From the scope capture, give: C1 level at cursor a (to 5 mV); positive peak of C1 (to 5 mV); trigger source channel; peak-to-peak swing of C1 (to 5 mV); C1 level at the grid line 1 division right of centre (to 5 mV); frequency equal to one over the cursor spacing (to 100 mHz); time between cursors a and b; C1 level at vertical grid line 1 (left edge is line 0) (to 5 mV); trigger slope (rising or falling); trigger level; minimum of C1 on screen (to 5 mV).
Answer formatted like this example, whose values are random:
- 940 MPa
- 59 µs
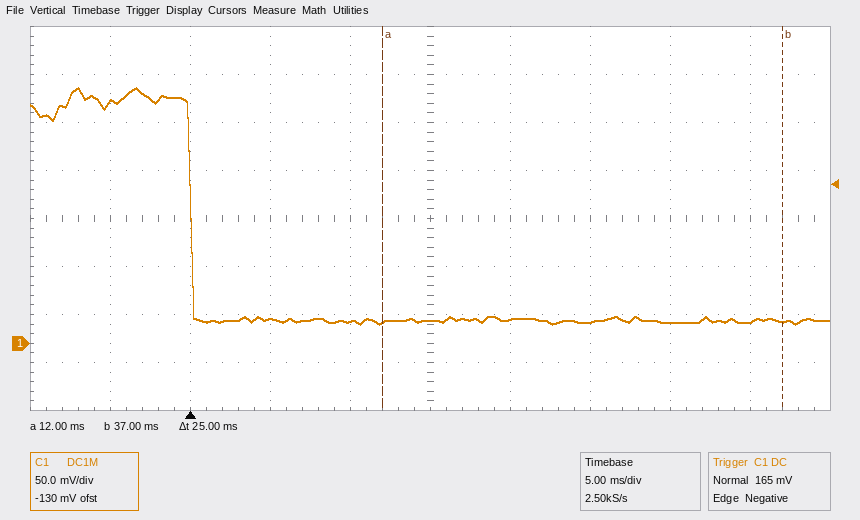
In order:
- 20 mV
- 265 mV
- C1
- 245 mV
- 25 mV
- 40.0 Hz
- 25 ms
- 250 mV
- falling
- 165 mV
- 20 mV
